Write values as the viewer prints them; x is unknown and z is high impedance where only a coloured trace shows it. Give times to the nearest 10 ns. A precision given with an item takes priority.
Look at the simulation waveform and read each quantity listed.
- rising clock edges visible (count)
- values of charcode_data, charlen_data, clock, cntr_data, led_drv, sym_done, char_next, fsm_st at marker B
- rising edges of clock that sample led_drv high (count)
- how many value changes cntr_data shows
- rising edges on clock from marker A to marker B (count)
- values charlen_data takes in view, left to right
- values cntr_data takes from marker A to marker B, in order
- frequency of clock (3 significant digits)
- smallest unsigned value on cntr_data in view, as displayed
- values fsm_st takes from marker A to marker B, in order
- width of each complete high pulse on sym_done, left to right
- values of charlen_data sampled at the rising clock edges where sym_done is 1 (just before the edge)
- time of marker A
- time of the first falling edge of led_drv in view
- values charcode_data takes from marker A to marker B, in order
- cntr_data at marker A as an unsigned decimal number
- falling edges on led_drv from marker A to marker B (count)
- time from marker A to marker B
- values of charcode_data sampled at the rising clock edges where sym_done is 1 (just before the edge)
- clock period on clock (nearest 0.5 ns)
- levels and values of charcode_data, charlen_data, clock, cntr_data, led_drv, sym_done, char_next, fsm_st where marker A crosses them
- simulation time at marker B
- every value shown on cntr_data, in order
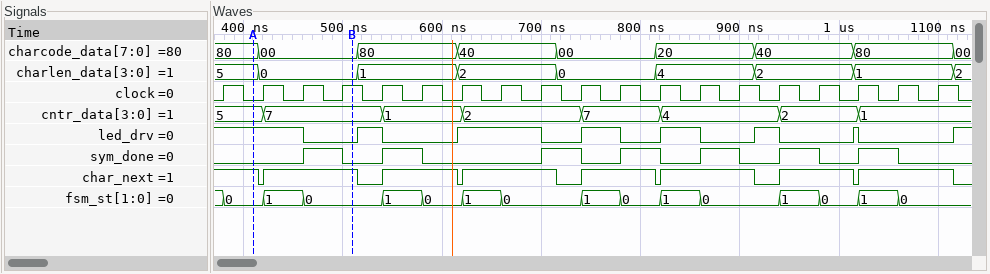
19
charcode_data=00, charlen_data=0, clock=1, cntr_data=7, led_drv=0, sym_done=0, char_next=1, fsm_st=0
11
7
3
5, 0, 1, 2, 0, 4, 2, 1, 2
5, 7
25.0 MHz
1
0, 1, 0
40 ns, 40 ns, 40 ns, 40 ns, 40 ns, 40 ns, 40 ns
0, 1, 0, 4, 4, 2, 1
410 ns
460 ns
80, 00
5
1
100 ns
00, 80, 00, 20, 20, 40, 80
40 ns
charcode_data=80, charlen_data=5, clock=0, cntr_data=5, led_drv=1, sym_done=0, char_next=1, fsm_st=0
510 ns
5, 7, 1, 2, 7, 4, 2, 1
